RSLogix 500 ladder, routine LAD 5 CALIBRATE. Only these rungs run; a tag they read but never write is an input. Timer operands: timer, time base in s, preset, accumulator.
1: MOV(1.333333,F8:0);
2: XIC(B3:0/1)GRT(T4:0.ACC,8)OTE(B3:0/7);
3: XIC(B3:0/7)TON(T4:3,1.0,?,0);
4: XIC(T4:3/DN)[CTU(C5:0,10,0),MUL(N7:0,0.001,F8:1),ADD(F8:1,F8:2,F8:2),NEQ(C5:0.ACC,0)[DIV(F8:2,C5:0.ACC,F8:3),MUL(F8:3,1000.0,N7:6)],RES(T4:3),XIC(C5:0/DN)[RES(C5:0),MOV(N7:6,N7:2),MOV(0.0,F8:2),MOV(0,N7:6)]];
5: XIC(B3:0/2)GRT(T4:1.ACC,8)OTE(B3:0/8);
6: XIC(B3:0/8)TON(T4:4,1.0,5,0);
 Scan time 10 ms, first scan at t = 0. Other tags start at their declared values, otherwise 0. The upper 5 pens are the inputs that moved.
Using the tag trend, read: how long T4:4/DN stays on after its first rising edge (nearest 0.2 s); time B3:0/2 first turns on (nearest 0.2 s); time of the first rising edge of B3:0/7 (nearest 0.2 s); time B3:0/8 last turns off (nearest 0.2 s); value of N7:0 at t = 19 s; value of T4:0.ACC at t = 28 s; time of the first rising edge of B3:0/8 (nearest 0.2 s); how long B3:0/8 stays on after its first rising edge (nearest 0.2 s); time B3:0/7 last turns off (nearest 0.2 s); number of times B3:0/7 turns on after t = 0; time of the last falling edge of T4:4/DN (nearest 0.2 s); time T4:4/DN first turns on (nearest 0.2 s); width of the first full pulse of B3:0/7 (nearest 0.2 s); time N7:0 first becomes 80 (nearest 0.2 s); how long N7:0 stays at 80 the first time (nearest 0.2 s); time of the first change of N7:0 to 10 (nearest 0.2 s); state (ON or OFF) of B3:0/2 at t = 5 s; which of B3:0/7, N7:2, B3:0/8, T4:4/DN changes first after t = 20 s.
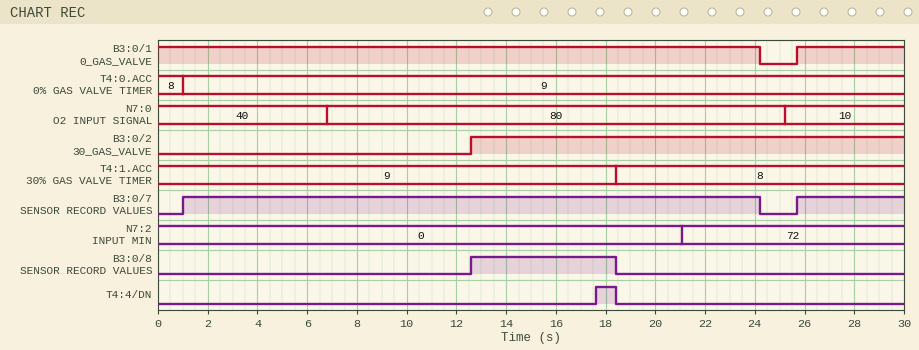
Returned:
0.8 s
12.6 s
1.0 s
18.4 s
80
9
12.6 s
5.8 s
24.2 s
2
18.4 s
17.6 s
23.2 s
6.8 s
18.4 s
25.2 s
OFF
N7:2
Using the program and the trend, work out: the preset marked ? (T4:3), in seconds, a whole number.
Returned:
2 s
